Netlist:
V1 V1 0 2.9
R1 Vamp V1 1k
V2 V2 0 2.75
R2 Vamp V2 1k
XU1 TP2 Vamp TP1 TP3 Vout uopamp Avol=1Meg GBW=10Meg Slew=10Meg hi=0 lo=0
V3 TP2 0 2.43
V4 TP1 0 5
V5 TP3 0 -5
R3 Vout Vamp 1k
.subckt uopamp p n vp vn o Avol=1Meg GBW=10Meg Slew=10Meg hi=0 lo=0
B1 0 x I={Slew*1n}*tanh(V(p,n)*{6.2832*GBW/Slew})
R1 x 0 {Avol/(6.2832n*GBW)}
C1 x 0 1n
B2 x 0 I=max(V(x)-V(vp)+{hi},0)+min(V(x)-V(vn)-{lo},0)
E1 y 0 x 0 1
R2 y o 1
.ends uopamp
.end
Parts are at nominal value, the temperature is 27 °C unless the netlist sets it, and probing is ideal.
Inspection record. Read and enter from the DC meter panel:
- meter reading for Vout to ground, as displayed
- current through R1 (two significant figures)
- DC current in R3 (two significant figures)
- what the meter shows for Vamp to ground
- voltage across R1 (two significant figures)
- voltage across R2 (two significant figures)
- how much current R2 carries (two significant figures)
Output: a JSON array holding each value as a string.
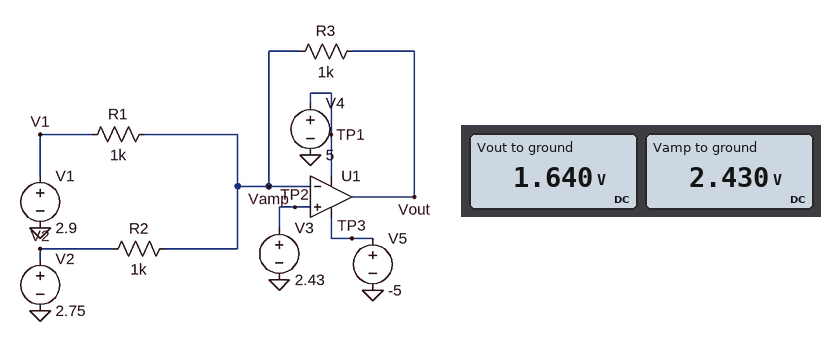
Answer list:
["1.640 V", "470 µA", "790 µA", "2.430 V", "470 mV", "320 mV", "320 µA"]
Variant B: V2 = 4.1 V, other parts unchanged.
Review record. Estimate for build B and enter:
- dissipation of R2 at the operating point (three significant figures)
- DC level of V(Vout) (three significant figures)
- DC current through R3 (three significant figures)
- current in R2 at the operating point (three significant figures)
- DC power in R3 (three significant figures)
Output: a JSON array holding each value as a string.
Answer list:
["2.79 mW", "290 mV", "2.14 mA", "1.67 mA", "4.58 mW"]
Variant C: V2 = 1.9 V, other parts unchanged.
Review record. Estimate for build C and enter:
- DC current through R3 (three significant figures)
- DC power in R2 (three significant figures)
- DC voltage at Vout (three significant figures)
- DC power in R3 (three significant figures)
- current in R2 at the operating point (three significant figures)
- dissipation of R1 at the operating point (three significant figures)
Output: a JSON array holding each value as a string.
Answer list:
["60.0 µA", "281 µW", "2.49 V", "3.60 µW", "530 µA", "221 µW"]
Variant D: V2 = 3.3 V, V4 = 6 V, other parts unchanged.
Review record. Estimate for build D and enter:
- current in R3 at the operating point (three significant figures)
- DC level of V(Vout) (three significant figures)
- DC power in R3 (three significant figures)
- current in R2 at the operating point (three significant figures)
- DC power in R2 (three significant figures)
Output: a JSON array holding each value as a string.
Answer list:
["1.34 mA", "1.09 V", "1.80 mW", "870 µA", "757 µW"]
